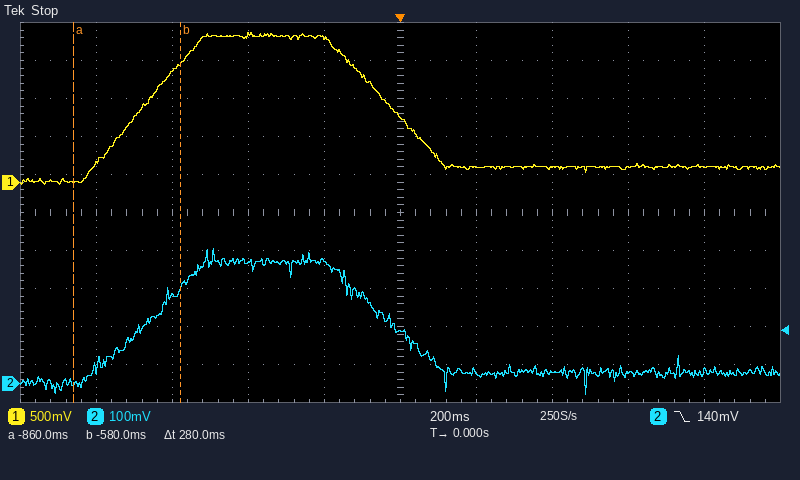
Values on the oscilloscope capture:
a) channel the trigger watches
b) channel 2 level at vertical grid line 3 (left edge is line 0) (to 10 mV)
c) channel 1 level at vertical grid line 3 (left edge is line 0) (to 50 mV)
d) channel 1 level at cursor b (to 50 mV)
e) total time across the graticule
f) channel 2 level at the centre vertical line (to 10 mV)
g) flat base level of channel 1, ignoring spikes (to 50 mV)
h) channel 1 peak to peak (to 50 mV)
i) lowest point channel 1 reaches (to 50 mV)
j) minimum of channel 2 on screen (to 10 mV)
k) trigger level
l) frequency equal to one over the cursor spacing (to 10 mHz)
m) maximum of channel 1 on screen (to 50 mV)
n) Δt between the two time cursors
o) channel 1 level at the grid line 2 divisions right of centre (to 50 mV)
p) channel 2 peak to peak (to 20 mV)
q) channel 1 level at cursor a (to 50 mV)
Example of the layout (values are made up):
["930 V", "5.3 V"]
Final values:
["channel 2", "320 mV", "1.95 V", "1.55 V", "2 s", "140 mV", "200 mV", "2.00 V", "-50 mV", "-30 mV", "140 mV", "3.57 Hz", "1.95 V", "280 ms", "200 mV", "380 mV", "0 mV"]
